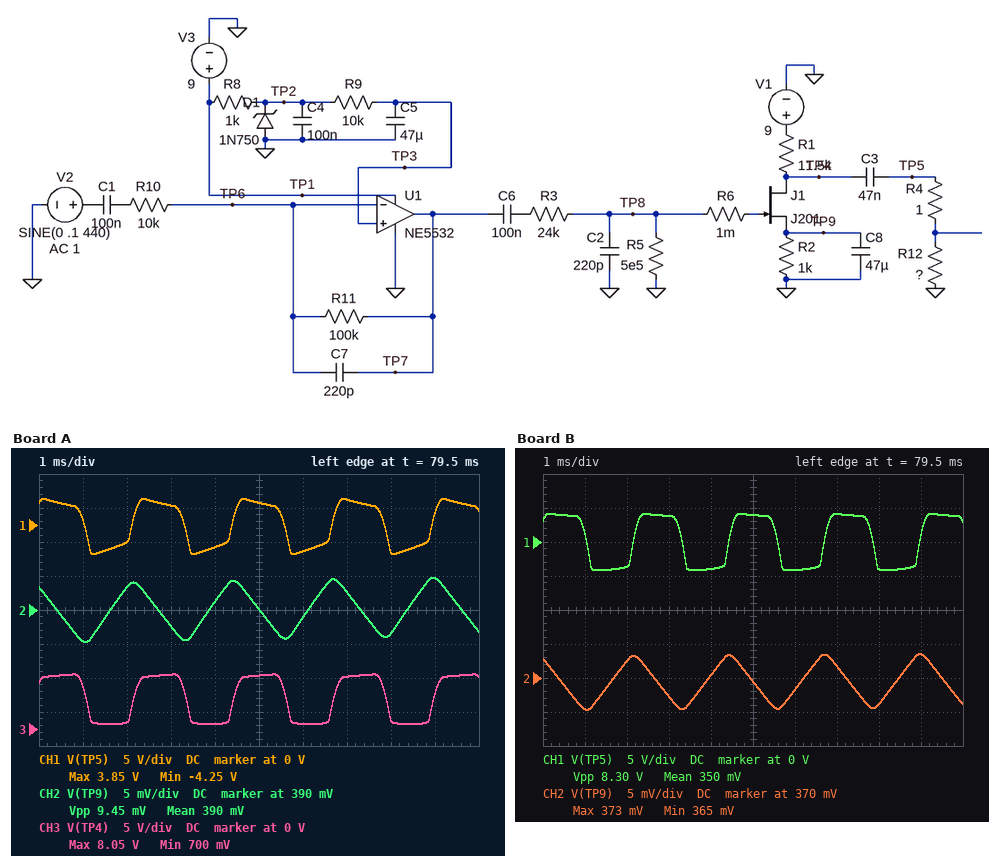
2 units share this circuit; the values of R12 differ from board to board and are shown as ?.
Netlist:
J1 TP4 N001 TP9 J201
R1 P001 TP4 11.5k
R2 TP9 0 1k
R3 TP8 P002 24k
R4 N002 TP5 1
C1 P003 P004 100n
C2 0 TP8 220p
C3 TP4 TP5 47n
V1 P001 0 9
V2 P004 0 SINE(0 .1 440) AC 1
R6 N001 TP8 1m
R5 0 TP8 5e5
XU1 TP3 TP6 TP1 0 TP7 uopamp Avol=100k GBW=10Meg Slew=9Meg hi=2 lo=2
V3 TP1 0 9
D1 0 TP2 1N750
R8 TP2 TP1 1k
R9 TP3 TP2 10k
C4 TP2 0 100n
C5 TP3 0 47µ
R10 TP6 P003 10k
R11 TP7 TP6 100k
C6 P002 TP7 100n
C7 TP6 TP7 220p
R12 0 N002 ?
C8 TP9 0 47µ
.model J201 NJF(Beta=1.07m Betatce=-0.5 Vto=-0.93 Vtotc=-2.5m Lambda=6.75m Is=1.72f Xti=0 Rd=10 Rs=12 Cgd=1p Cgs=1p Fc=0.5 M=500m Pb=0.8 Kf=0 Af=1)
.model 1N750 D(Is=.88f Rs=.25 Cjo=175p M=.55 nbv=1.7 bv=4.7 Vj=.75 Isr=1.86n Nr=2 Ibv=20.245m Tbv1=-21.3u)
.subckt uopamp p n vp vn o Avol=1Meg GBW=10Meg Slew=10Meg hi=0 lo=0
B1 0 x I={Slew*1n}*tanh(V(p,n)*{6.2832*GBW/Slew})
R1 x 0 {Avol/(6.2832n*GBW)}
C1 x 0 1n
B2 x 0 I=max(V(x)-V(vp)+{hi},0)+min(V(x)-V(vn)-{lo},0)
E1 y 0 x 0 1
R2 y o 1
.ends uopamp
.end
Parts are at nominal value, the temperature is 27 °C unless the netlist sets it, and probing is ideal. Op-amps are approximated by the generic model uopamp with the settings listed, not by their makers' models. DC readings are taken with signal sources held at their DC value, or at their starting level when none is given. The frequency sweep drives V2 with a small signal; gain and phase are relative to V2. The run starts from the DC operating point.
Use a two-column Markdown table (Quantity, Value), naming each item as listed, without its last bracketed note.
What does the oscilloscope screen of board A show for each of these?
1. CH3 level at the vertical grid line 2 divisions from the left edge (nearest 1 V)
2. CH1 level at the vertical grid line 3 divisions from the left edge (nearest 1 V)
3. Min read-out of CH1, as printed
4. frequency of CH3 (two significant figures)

| Quantity | Value |
|---|---|
| CH3 level at the vertical grid line 2 divisions from the left edge | 1 V |
| CH1 level at the vertical grid line 3 divisions from the left edge | 3 V |
| Min read-out of CH1, as printed | -4.25 V |
| frequency of CH3 | 440 Hz |
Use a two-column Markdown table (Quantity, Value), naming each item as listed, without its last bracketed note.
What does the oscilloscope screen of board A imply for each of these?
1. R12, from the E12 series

| Quantity | Value |
|---|---|
| R12, from the E12 series | 33 kΩ |
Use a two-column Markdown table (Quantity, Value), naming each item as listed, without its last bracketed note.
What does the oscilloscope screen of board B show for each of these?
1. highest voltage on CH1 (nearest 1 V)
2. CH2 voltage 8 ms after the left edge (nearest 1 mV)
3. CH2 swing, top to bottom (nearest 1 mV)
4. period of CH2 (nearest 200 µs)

| Quantity | Value |
|---|---|
| highest voltage on CH1 | 4 V |
| CH2 voltage 8 ms after the left edge | 366 mV |
| CH2 swing, top to bottom | 8 mV |
| period of CH2 | 2.2 ms |
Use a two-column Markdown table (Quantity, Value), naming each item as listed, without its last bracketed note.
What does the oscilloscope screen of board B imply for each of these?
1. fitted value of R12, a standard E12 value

| Quantity | Value |
|---|---|
| fitted value of R12, a standard E12 value | 150 kΩ |
